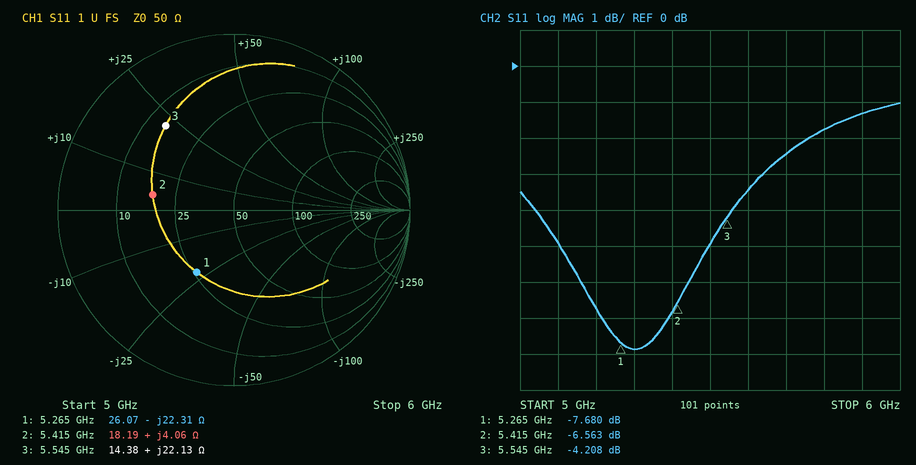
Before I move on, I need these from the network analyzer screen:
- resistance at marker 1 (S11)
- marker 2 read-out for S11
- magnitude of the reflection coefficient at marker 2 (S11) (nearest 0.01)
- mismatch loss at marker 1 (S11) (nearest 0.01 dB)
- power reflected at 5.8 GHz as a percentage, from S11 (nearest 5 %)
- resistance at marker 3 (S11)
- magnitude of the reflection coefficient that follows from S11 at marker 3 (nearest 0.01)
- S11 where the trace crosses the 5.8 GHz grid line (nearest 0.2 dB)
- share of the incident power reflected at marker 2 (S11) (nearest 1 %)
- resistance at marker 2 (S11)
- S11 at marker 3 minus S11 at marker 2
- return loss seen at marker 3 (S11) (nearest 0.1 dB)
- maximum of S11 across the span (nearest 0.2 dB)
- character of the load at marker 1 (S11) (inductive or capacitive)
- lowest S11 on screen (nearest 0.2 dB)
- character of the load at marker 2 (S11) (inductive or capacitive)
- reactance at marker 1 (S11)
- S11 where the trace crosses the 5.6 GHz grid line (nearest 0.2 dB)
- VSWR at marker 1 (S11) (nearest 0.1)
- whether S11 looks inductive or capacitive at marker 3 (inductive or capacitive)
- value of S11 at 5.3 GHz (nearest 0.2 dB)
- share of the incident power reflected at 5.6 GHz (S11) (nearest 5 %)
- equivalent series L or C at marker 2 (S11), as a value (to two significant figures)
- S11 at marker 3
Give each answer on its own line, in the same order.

26.07 Ω
-6.563 dB
0.47
0.81 dB
65 %
14.38 Ω
0.62
-1.8 dB
22 %
18.19 Ω
2.355 dB
4.2 dB
-1.0 dB
capacitive
-7.8 dB
inductive
-22.31 Ω
-3.4 dB
2.4
inductive
-7.8 dB
45 %
120 pH
-4.208 dB
